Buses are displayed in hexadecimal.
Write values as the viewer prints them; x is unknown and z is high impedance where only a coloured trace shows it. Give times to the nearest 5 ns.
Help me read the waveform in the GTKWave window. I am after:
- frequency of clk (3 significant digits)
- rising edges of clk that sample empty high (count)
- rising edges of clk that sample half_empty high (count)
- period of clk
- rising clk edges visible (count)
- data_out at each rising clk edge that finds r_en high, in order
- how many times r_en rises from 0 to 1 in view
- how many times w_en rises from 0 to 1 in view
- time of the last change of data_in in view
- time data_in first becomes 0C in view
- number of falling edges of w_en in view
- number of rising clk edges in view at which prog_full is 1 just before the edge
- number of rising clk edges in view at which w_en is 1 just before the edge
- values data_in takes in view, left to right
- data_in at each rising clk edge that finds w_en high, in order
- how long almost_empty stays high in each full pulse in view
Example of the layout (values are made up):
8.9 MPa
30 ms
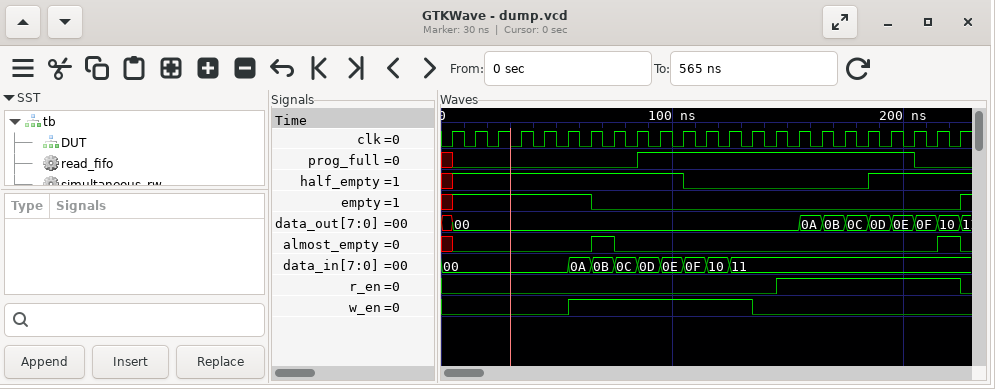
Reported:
100 MHz
6
14
10 ns
23
00, 0A, 0B, 0C, 0D, 0E, 0F, 10
1
1
125 ns
75 ns
1
12
8
00, 0A, 0B, 0C, 0D, 0E, 0F, 10, 11
0A, 0B, 0C, 0D, 0E, 0F, 10, 11
10 ns, 10 ns
